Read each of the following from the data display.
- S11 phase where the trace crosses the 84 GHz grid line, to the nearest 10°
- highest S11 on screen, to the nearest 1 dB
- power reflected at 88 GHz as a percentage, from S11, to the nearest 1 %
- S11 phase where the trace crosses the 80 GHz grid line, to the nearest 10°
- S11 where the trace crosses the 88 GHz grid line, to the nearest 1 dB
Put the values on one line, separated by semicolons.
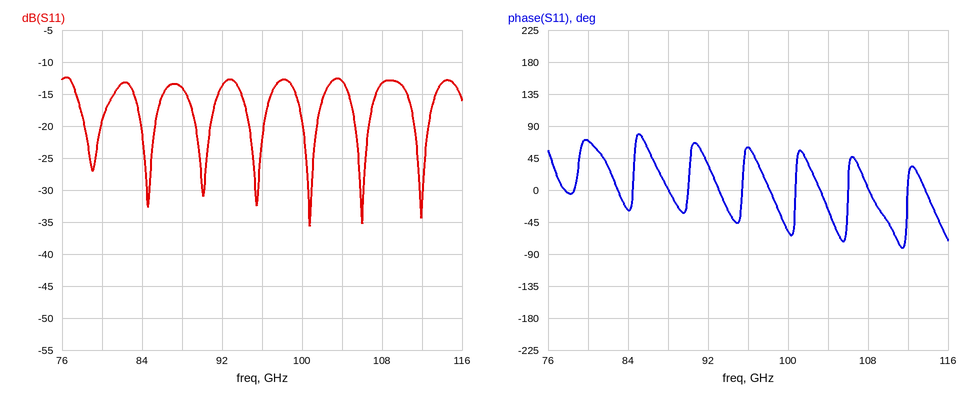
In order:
-30°; -12 dB; 4 %; 70°; -14 dB
